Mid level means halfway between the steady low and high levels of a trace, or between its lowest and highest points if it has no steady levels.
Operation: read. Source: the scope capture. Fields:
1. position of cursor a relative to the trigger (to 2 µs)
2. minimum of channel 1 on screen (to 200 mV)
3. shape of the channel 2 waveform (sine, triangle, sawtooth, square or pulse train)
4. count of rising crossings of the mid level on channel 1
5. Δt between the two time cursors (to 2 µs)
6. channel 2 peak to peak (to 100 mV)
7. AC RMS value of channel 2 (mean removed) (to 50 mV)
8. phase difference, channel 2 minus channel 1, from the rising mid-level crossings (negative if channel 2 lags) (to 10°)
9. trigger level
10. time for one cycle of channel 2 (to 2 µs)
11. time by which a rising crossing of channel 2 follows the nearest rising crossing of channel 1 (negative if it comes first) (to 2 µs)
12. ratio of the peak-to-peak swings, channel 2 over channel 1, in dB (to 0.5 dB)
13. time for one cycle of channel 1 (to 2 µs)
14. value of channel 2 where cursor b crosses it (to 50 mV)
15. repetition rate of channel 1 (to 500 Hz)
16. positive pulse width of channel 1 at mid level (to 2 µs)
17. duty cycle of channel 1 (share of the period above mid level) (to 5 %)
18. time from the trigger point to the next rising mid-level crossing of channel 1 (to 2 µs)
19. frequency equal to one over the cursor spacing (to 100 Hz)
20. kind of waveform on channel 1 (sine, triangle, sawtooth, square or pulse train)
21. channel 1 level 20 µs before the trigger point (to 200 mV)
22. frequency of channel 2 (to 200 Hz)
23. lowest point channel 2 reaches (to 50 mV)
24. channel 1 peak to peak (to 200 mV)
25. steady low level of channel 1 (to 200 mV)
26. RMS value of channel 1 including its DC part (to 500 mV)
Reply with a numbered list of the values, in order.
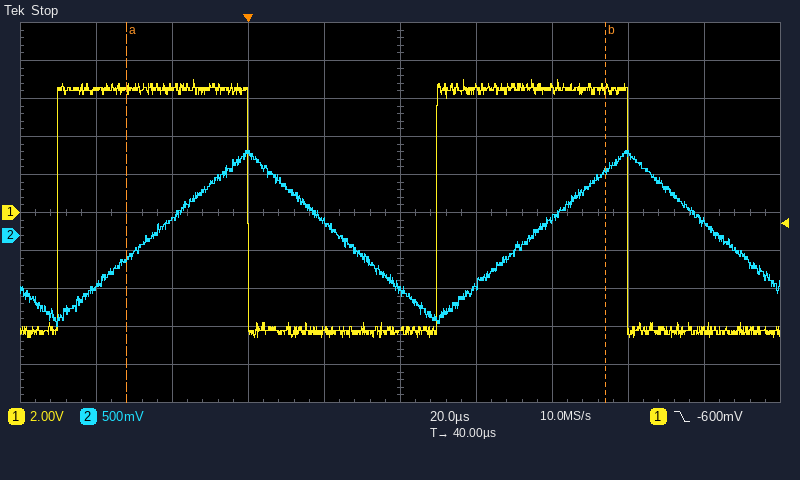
1. -32 µs
2. -6.6 V
3. triangle
4. 2
5. 126 µs
6. 2.30 V
7. 650 mV
8. -90°
9. -600 mV
10. 100 µs
11. +24 µs
12. -15.5 dB
13. 100 µs
14. 850 mV
15. 10.0 kHz
16. 50 µs
17. 50 %
18. 50 µs
19. 7.9 kHz
20. square
21. 6.6 V
22. 10.0 kHz
23. -1.20 V
24. 13.6 V
25. -6.2 V
26. 6.5 V
